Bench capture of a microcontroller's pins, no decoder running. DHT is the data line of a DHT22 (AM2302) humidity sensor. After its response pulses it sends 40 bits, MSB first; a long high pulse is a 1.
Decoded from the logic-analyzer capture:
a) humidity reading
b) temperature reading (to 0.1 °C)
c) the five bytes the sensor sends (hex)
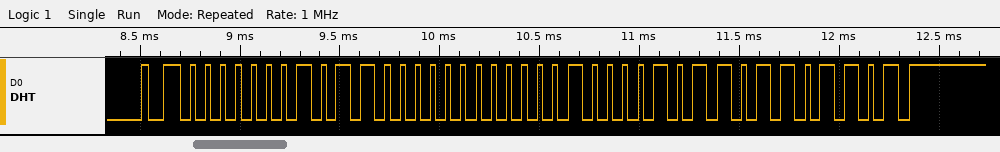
35.2 %
26.7 °C
01 60 01 0B 6D
